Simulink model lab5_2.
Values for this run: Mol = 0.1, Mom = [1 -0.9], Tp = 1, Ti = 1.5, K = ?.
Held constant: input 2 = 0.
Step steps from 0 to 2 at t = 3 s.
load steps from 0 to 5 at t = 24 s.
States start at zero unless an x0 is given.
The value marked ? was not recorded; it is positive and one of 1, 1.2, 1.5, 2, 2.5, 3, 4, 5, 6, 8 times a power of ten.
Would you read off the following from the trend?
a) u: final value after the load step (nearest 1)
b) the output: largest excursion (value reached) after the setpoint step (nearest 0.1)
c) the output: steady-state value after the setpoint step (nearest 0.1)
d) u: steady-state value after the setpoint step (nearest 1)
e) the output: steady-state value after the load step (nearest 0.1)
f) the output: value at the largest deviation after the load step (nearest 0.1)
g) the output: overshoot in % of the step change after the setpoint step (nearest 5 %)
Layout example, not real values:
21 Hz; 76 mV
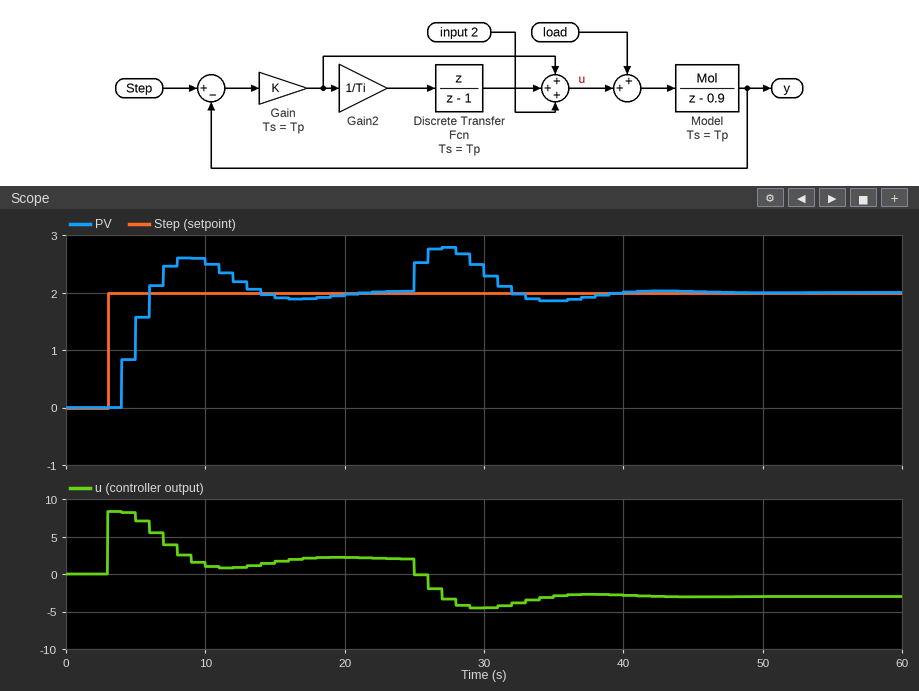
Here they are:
-3; 2.6; 2.0; 2; 2.0; 2.8; 30 %
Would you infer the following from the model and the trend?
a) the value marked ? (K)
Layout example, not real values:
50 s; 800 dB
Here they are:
2.5
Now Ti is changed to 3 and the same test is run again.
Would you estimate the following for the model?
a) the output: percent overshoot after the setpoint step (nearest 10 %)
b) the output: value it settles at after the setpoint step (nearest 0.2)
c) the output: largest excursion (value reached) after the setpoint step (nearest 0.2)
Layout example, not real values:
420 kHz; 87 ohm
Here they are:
20 %; 2.0; 2.4
